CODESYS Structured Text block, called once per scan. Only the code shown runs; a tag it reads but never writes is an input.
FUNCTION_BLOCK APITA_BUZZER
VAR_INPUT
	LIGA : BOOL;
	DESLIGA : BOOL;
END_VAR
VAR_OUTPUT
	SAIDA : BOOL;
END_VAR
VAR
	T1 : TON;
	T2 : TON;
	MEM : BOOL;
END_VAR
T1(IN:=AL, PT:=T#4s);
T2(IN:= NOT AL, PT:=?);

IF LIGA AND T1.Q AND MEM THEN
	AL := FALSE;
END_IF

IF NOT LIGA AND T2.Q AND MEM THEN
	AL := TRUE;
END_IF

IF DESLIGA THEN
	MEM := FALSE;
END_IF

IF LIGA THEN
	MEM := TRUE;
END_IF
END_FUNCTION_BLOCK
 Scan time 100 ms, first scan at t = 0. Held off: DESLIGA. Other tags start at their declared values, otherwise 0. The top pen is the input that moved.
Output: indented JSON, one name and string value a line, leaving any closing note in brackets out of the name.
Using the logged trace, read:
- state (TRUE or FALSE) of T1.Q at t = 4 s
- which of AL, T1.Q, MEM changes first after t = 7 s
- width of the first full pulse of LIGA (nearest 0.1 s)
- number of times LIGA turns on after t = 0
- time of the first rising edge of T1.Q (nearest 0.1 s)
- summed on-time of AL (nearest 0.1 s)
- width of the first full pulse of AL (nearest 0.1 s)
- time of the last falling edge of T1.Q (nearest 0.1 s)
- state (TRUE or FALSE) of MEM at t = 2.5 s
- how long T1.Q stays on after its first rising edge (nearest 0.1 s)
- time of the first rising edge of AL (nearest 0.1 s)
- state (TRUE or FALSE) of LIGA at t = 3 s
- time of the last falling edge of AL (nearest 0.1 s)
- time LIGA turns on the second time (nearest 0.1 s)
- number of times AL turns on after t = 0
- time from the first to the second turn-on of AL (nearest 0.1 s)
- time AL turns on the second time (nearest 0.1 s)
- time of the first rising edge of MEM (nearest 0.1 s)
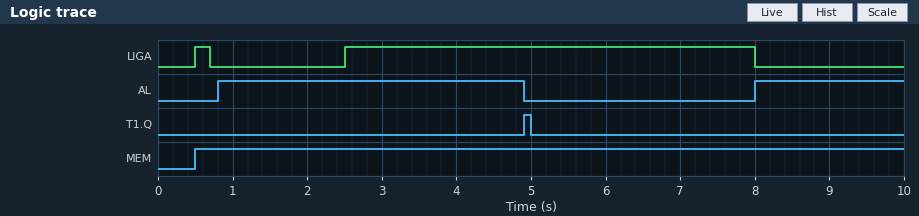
{
  "state (TRUE or FALSE) of T1.Q at t = 4 s": "FALSE",
  "which of AL, T1.Q, MEM changes first after t = 7 s": "AL",
  "width of the first full pulse of LIGA": "0.2 s",
  "number of times LIGA turns on after t = 0": "2",
  "time of the first rising edge of T1.Q": "4.9 s",
  "summed on-time of AL": "6.1 s",
  "width of the first full pulse of AL": "4.1 s",
  "time of the last falling edge of T1.Q": "5.0 s",
  "state (TRUE or FALSE) of MEM at t = 2.5 s": "TRUE",
  "how long T1.Q stays on after its first rising edge": "0.1 s",
  "time of the first rising edge of AL": "0.8 s",
  "state (TRUE or FALSE) of LIGA at t = 3 s": "TRUE",
  "time of the last falling edge of AL": "4.9 s",
  "time LIGA turns on the second time": "2.5 s",
  "number of times AL turns on after t = 0": "2",
  "time from the first to the second turn-on of AL": "7.2 s",
  "time AL turns on the second time": "8.0 s",
  "time of the first rising edge of MEM": "0.5 s"
}
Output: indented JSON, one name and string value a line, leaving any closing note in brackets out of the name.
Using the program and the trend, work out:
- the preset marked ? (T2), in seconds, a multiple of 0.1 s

{
  "the preset marked ? (T2), in seconds, a multiple of 0.1 s": "0.8 s"
}
